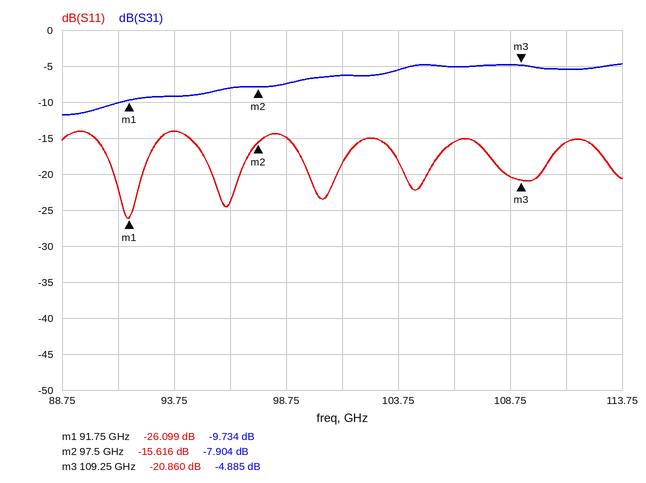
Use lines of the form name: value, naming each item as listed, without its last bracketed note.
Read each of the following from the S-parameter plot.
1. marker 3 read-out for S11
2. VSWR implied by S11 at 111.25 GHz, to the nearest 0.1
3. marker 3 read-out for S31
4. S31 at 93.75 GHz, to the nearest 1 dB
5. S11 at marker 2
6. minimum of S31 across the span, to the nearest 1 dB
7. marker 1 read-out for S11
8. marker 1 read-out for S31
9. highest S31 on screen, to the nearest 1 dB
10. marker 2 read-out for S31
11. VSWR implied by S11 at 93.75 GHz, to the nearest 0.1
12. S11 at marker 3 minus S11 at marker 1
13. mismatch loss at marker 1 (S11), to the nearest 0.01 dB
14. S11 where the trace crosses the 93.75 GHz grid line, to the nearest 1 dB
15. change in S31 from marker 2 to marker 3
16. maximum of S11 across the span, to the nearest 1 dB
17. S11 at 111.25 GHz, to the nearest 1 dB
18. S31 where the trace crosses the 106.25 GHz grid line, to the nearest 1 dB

marker 3 read-out for S11: -20.860 dB
VSWR implied by S11 at 111.25 GHz, to the nearest 0.1: 1.4
marker 3 read-out for S31: -4.885 dB
S31 at 93.75 GHz, to the nearest 1 dB: -9 dB
S11 at marker 2: -15.616 dB
minimum of S31 across the span, to the nearest 1 dB: -12 dB
marker 1 read-out for S11: -26.099 dB
marker 1 read-out for S31: -9.734 dB
highest S31 on screen, to the nearest 1 dB: -5 dB
marker 2 read-out for S31: -7.904 dB
VSWR implied by S11 at 93.75 GHz, to the nearest 0.1: 1.5
S11 at marker 3 minus S11 at marker 1: 5.239 dB
mismatch loss at marker 1 (S11), to the nearest 0.01 dB: 0.01 dB
S11 where the trace crosses the 93.75 GHz grid line, to the nearest 1 dB: -14 dB
change in S31 from marker 2 to marker 3: 3.019 dB
maximum of S11 across the span, to the nearest 1 dB: -14 dB
S11 at 111.25 GHz, to the nearest 1 dB: -16 dB
S31 where the trace crosses the 106.25 GHz grid line, to the nearest 1 dB: -5 dB
